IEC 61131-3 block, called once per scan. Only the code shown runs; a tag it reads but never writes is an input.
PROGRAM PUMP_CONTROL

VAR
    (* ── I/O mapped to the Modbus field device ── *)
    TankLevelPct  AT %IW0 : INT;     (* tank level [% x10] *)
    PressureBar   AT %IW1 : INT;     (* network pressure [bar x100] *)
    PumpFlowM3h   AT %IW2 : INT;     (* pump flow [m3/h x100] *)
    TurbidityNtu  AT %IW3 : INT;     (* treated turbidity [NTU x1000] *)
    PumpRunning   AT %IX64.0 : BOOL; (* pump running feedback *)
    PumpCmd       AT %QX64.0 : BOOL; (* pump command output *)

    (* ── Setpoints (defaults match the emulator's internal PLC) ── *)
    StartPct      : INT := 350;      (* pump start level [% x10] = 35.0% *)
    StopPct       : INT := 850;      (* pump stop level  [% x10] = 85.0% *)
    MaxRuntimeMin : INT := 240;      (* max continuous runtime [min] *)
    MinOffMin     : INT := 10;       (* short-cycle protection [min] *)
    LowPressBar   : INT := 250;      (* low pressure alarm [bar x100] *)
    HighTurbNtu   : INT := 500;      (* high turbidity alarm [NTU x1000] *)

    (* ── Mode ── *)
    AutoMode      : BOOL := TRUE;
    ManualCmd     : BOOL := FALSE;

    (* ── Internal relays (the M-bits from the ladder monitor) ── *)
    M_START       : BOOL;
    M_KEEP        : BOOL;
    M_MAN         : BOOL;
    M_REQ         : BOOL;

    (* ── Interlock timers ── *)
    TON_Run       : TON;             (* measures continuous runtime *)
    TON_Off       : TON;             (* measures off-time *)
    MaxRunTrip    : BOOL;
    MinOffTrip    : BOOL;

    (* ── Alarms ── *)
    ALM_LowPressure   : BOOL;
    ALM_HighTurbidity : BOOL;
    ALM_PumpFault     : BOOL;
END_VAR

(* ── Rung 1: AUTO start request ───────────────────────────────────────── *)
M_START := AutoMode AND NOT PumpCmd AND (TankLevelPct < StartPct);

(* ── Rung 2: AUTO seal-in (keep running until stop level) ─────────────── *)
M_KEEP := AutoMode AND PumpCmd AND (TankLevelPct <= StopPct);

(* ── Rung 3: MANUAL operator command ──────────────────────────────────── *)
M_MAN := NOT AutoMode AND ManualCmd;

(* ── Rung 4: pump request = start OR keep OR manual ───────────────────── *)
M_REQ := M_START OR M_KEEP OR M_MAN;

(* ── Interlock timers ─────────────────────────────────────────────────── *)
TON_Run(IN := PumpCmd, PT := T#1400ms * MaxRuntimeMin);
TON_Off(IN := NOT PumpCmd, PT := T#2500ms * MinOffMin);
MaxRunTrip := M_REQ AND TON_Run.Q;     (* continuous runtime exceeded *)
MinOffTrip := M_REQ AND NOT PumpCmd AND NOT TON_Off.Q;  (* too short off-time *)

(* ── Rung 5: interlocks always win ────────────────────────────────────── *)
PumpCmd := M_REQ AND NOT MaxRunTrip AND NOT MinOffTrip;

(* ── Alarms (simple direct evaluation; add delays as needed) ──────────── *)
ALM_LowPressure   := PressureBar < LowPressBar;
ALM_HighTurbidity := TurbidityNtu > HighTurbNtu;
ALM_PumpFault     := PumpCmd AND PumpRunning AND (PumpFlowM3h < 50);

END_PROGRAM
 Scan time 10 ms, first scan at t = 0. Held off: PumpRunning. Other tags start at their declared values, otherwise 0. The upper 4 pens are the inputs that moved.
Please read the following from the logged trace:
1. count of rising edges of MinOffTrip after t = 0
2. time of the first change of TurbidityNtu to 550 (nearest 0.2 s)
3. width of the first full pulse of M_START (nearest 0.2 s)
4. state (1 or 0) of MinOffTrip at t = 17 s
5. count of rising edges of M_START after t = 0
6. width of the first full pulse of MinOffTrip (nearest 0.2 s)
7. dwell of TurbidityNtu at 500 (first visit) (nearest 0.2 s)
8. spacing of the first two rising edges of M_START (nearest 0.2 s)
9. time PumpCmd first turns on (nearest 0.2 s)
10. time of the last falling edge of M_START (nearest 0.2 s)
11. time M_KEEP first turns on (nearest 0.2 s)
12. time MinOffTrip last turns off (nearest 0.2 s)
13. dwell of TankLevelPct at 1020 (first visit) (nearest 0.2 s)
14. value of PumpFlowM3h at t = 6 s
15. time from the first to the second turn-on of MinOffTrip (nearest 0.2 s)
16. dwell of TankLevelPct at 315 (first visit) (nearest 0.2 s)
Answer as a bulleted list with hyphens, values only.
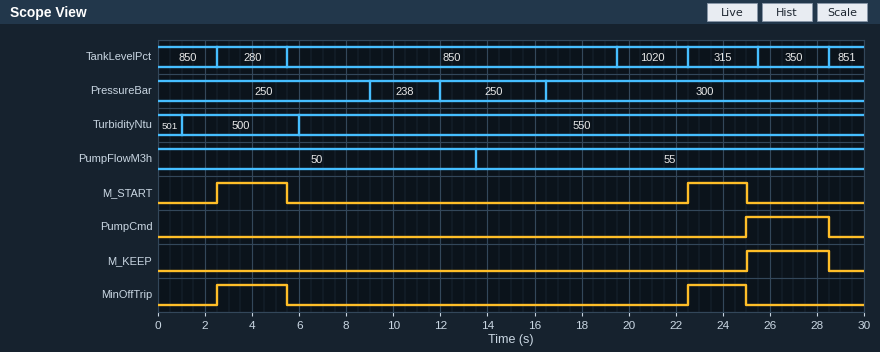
- 2
- 6.0 s
- 3.0 s
- 0
- 2
- 3.0 s
- 5.0 s
- 20.0 s
- 25.0 s
- 25.0 s
- 25.0 s
- 25.0 s
- 3.0 s
- 50
- 20.0 s
- 3.0 s
